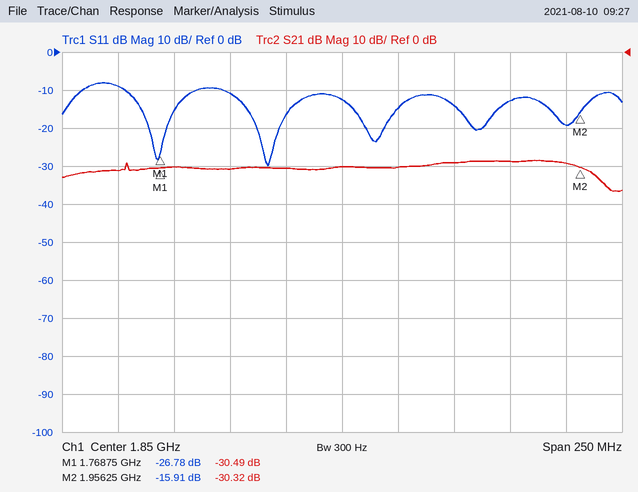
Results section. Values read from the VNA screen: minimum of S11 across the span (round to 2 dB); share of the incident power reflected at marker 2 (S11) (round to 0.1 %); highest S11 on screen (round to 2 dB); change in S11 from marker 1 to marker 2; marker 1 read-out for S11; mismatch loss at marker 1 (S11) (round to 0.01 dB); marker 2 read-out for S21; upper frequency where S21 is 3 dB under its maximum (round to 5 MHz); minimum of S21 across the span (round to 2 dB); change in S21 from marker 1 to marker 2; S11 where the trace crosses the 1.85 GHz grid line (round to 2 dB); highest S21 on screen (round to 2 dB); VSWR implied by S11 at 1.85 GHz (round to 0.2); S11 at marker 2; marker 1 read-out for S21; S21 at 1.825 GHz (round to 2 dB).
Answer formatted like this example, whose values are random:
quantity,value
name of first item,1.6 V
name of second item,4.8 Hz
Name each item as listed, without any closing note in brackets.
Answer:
quantity,value
minimum of S11 across the span,-30 dB
share of the incident power reflected at marker 2 (S11),2.6 %
highest S11 on screen,-8 dB
change in S11 from marker 1 to marker 2,10.87 dB
marker 1 read-out for S11,-26.78 dB
mismatch loss at marker 1 (S11),0.01 dB
marker 2 read-out for S21,-30.32 dB
upper frequency where S21 is 3 dB under its maximum,1.960 GHz
minimum of S21 across the span,-36 dB
change in S21 from marker 1 to marker 2,0.17 dB
S11 where the trace crosses the 1.85 GHz grid line,-12 dB
highest S21 on screen,-28 dB
VSWR implied by S11 at 1.85 GHz,1.6
S11 at marker 2,-15.91 dB
marker 1 read-out for S21,-30.49 dB
S21 at 1.825 GHz,-30 dB
